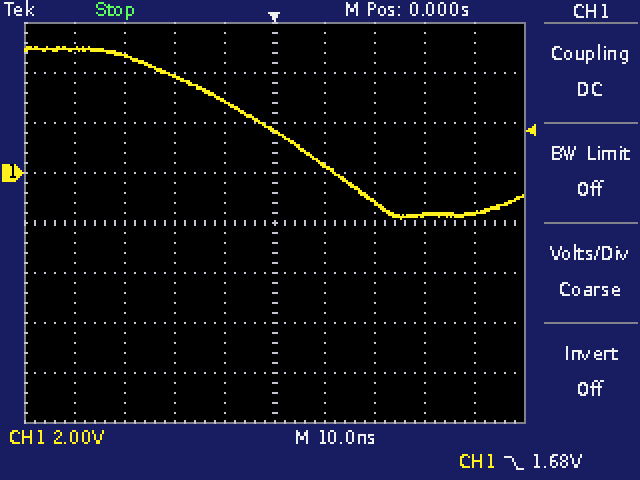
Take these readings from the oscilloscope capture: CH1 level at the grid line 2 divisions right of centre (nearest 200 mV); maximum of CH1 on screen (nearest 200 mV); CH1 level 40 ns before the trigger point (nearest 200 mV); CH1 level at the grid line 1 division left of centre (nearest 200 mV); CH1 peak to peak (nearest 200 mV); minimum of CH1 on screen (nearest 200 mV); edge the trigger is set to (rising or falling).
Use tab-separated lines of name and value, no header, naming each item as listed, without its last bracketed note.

CH1 level at the grid line 2 divisions right of centre	-1.2 V
maximum of CH1 on screen	5.0 V
CH1 level 40 ns before the trigger point	5.0 V
CH1 level at the grid line 1 division left of centre	2.8 V
CH1 peak to peak	6.8 V
minimum of CH1 on screen	-1.8 V
edge the trigger is set to	falling
